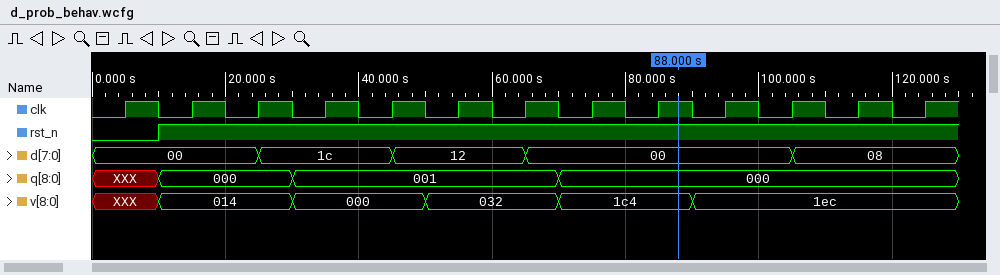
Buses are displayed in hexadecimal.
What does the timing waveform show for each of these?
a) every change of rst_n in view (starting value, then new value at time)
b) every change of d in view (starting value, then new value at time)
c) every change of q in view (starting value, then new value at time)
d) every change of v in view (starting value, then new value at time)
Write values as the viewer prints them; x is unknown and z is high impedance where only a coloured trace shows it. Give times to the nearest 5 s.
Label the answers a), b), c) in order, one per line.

a) 0, 1 at 10 s
b) 00, 1c at 25 s, 12 at 45 s, 00 at 65 s, 08 at 105 s
c) XXX, 000 at 10 s, 001 at 30 s, 000 at 70 s
d) XXX, 014 at 10 s, 000 at 30 s, 032 at 50 s, 1c4 at 70 s, 1ec at 90 s
